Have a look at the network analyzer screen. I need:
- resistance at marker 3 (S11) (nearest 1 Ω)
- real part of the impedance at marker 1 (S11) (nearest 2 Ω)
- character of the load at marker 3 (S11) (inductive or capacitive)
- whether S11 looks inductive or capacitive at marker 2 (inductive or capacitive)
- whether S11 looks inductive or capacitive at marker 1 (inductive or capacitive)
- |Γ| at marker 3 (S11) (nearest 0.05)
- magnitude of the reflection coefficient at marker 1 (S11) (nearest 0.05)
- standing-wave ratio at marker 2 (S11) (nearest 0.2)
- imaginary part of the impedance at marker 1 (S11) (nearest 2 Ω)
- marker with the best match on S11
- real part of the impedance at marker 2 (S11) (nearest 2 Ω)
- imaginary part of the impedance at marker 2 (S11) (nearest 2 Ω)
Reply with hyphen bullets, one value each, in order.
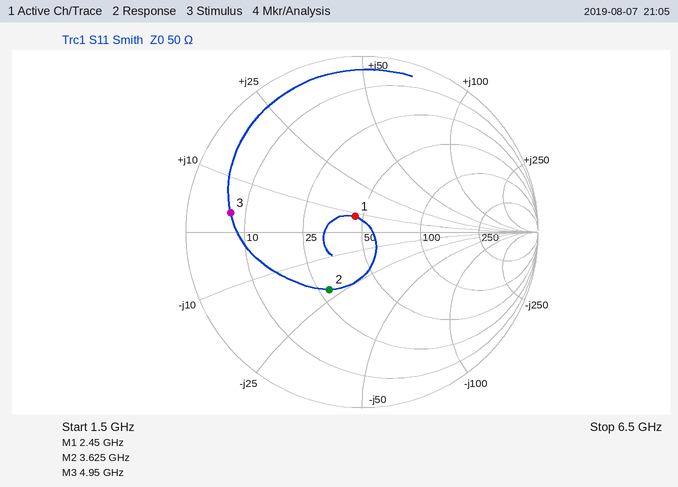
- 7 Ω
- 46 Ω
- inductive
- capacitive
- inductive
- 0.75
- 0.10
- 2.2
- +8 Ω
- marker 1
- 28 Ω
- -22 Ω
